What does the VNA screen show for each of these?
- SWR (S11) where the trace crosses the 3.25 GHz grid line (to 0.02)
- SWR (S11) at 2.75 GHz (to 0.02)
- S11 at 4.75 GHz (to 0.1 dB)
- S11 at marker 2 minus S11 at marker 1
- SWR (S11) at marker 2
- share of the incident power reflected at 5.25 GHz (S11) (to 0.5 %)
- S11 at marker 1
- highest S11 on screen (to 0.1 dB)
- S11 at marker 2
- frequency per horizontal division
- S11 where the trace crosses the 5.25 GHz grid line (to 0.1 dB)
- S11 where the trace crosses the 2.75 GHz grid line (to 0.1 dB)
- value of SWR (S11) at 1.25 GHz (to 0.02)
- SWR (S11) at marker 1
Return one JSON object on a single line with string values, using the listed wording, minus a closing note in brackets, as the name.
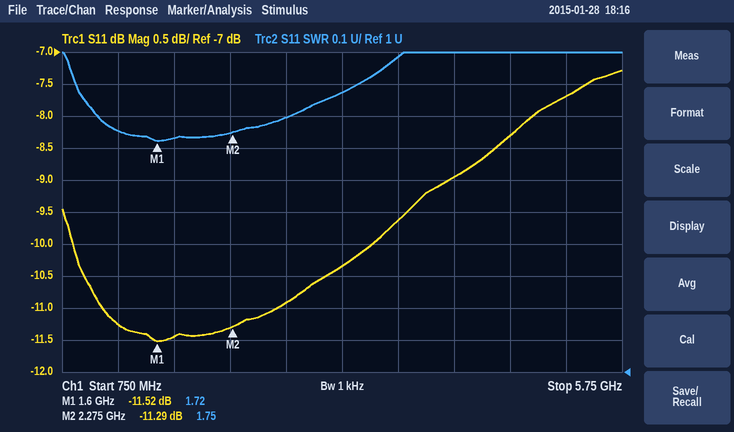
{"SWR (S11) where the trace crosses the 3.25 GHz grid line": "1.88", "SWR (S11) at 2.75 GHz": "1.80", "S11 at 4.75 GHz": "-8.3 dB", "S11 at marker 2 minus S11 at marker 1": "0.23 dB", "SWR (S11) at marker 2": "1.75", "share of the incident power reflected at 5.25 GHz (S11)": "17.0 %", "S11 at marker 1": "-11.52 dB", "highest S11 on screen": "-7.3 dB", "S11 at marker 2": "-11.29 dB", "frequency per horizontal division": "500 MHz", "S11 where the trace crosses the 5.25 GHz grid line": "-7.7 dB", "S11 where the trace crosses the 2.75 GHz grid line": "-10.9 dB", "value of SWR (S11) at 1.25 GHz": "1.76", "SWR (S11) at marker 1": "1.72"}
